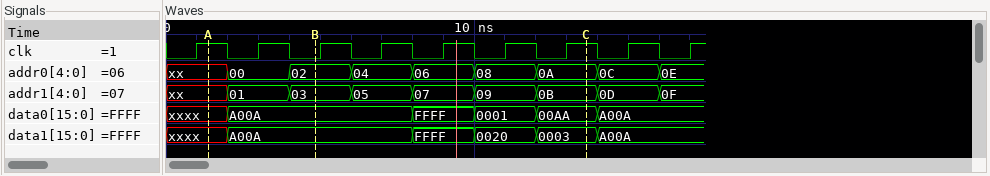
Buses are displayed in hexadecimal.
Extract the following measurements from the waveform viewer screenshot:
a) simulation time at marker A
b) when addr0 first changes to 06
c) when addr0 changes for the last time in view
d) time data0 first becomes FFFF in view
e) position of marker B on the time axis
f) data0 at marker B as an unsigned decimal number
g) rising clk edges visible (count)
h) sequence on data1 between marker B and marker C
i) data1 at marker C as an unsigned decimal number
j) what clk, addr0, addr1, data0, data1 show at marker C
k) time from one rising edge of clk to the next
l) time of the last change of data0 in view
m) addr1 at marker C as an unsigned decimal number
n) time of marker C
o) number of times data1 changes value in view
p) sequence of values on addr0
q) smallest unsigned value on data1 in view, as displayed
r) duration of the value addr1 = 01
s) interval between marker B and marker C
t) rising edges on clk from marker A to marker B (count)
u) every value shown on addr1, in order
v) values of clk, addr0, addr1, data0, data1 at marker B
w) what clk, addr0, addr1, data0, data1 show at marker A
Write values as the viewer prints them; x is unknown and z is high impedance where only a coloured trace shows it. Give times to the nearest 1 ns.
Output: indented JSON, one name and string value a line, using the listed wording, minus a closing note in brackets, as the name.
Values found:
{
  "simulation time at marker A": "1 ns",
  "when addr0 first changes to 06": "8 ns",
  "when addr0 changes for the last time in view": "16 ns",
  "time data0 first becomes FFFF in view": "8 ns",
  "position of marker B on the time axis": "5 ns",
  "data0 at marker B as an unsigned decimal number": "40970",
  "rising clk edges visible": "9",
  "sequence on data1 between marker B and marker C": "A00A, FFFF, 0020, 0003",
  "data1 at marker C as an unsigned decimal number": "3",
  "what clk, addr0, addr1, data0, data1 show at marker C": "clk=1, addr0=0A, addr1=0B, data0=00AA, data1=0003",
  "time from one rising edge of clk to the next": "2 ns",
  "time of the last change of data0 in view": "14 ns",
  "addr1 at marker C as an unsigned decimal number": "11",
  "time of marker C": "14 ns",
  "number of times data1 changes value in view": "5",
  "sequence of values on addr0": "xx, 00, 02, 04, 06, 08, 0A, 0C, 0E",
  "smallest unsigned value on data1 in view, as displayed": "0003",
  "duration of the value addr1 = 01": "2 ns",
  "interval between marker B and marker C": "9 ns",
  "rising edges on clk from marker A to marker B": "1",
  "every value shown on addr1, in order": "xx, 01, 03, 05, 07, 09, 0B, 0D, 0F",
  "values of clk, addr0, addr1, data0, data1 at marker B": "clk=0, addr0=02, addr1=03, data0=A00A, data1=A00A",
  "what clk, addr0, addr1, data0, data1 show at marker A": "clk=1, addr0=xx, addr1=xx, data0=xxxx, data1=xxxx"
}
